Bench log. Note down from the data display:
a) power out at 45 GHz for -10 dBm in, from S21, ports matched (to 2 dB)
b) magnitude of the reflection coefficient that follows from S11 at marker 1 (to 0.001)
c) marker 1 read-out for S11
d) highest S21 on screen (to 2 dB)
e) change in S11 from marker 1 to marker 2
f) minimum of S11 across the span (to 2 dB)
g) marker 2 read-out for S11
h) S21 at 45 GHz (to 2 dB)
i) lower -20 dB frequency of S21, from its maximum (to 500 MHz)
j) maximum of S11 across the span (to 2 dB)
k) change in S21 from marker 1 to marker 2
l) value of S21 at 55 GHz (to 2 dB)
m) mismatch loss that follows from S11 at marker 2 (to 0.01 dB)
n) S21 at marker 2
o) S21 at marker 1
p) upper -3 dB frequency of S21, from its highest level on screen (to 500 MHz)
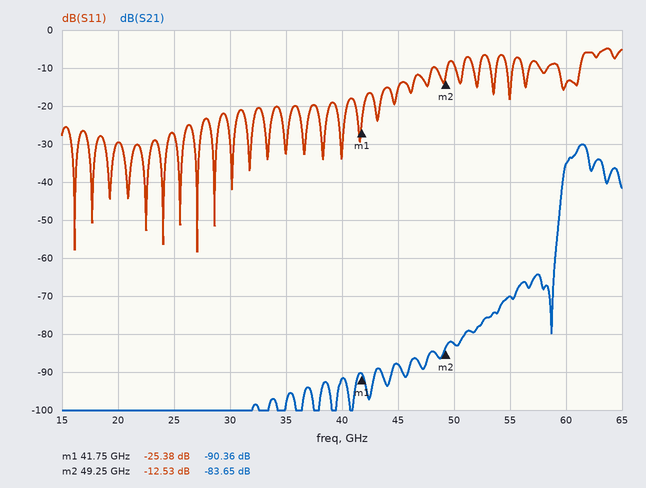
-98 dBm
0.054
-25.38 dB
-30 dB
12.85 dB
-58 dB
-12.53 dB
-88 dB
59.5 GHz
-4 dB
6.71 dB
-70 dB
0.25 dB
-83.65 dB
-90.36 dB
62.0 GHz
